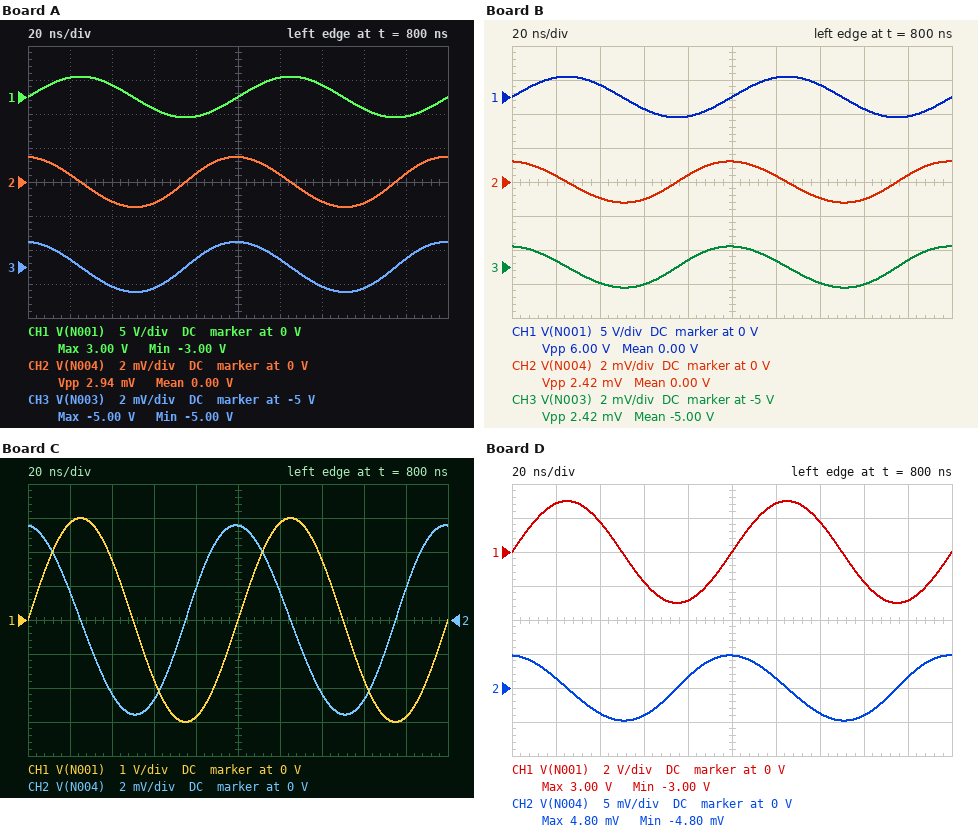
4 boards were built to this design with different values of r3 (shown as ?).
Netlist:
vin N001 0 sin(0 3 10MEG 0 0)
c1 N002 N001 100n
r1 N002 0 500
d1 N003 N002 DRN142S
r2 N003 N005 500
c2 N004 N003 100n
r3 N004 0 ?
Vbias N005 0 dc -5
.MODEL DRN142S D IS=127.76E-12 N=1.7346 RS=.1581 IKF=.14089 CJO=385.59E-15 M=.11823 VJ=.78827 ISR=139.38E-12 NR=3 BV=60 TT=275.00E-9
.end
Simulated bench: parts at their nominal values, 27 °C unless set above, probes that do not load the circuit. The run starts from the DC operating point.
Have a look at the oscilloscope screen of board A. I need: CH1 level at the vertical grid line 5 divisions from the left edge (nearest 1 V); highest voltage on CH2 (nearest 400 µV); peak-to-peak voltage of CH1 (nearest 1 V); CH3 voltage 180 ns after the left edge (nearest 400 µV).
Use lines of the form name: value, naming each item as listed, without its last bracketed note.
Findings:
CH1 level at the vertical grid line 5 divisions from the left edge: 0 V
highest voltage on CH2: 1.6 mV
peak-to-peak voltage of CH1: 6 V
CH3 voltage 180 ns after the left edge: -4.9996 V
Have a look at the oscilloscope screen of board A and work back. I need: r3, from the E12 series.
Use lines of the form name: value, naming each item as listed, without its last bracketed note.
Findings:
r3, from the E12 series: 27 Ω
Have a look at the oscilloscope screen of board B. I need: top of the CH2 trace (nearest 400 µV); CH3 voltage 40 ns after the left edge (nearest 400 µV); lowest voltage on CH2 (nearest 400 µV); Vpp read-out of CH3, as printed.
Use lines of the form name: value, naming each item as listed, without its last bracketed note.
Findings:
top of the CH2 trace: 1.2 mV
CH3 voltage 40 ns after the left edge: -5.0008 V
lowest voltage on CH2: -1.2 mV
Vpp read-out of CH3, as printed: 2.42 mV
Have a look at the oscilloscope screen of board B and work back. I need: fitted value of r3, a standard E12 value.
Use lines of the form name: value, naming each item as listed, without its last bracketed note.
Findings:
fitted value of r3, a standard E12 value: 22 Ω
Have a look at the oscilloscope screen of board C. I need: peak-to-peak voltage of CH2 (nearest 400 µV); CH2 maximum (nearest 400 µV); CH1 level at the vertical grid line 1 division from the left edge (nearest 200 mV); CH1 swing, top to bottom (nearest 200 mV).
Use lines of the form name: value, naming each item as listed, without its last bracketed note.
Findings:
peak-to-peak voltage of CH2: 11.2 mV
CH2 maximum: 5.6 mV
CH1 level at the vertical grid line 1 division from the left edge: 2.8 V
CH1 swing, top to bottom: 6.0 V
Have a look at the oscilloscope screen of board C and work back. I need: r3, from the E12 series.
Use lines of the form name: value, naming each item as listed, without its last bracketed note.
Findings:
r3, from the E12 series: 120 Ω
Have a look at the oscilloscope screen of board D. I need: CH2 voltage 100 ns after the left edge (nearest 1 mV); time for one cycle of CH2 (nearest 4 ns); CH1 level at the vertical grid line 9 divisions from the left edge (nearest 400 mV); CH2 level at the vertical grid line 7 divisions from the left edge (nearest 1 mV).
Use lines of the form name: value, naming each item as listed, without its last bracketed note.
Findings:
CH2 voltage 100 ns after the left edge: 5 mV
time for one cycle of CH2: 100 ns
CH1 level at the vertical grid line 9 divisions from the left edge: -2.8 V
CH2 level at the vertical grid line 7 divisions from the left edge: -4 mV
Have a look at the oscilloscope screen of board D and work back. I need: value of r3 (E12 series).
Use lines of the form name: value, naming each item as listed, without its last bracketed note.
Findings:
value of r3: 100 Ω
